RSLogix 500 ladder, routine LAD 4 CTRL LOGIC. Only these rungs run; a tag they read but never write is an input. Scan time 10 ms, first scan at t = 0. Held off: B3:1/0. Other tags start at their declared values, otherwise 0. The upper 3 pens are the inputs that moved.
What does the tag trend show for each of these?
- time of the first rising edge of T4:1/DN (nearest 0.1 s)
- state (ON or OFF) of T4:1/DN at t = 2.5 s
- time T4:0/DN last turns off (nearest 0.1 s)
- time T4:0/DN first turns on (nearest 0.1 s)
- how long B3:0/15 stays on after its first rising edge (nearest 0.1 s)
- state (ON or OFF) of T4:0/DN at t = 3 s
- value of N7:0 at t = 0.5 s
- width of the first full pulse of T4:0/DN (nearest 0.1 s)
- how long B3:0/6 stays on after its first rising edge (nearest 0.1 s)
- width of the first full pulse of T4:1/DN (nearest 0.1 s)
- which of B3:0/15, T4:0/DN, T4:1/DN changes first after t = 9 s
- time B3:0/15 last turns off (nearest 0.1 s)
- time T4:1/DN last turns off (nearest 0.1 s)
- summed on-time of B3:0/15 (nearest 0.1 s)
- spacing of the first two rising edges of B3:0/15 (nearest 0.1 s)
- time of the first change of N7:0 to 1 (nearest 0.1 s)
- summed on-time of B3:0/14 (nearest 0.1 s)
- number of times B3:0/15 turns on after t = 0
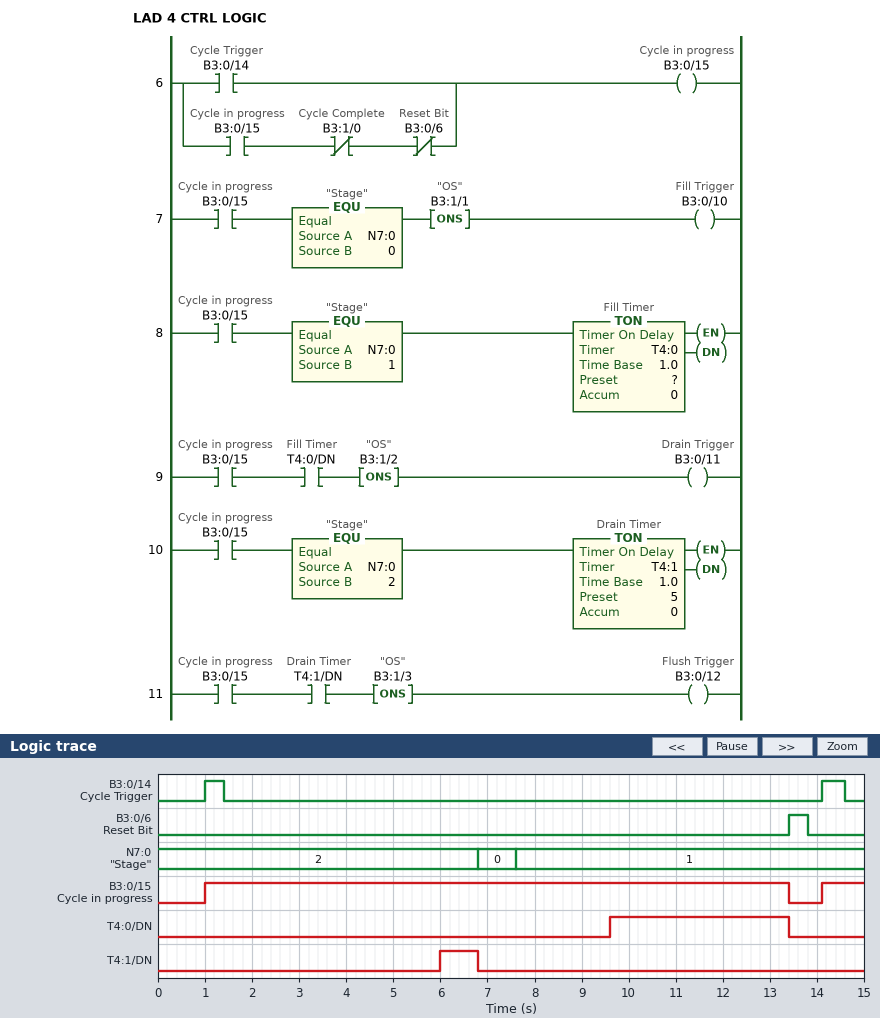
6.0 s
OFF
13.4 s
9.6 s
12.4 s
OFF
2
3.8 s
0.4 s
0.8 s
T4:0/DN
13.4 s
6.8 s
13.3 s
13.1 s
7.6 s
0.9 s
2
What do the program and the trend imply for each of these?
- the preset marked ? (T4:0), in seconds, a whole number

2 s
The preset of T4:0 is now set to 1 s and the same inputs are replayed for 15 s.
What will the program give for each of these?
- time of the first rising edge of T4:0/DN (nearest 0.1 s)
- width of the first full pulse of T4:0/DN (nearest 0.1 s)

8.6 s
4.8 s
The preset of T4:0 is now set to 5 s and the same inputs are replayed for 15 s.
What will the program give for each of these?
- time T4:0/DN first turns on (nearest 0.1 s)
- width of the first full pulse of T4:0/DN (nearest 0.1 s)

12.6 s
0.8 s
